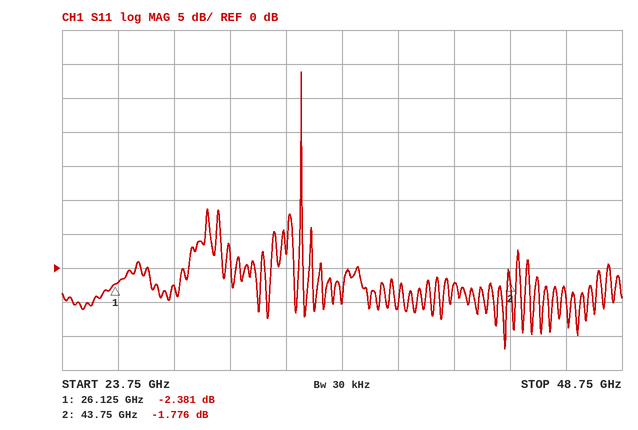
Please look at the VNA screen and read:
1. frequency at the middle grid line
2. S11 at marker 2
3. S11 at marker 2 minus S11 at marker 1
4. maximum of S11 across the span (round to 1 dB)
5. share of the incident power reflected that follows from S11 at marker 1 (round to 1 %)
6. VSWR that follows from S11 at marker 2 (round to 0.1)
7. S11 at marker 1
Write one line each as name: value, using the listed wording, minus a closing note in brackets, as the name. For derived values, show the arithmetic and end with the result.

frequency at the middle grid line: 36.25 GHz
S11 at marker 2: -1.776 dB
S11 at marker 2 minus S11 at marker 1: -1.776 − (-2.381) = 0.605 dB
maximum of S11 across the span: 29 dB
share of the incident power reflected that follows from S11 at marker 1: 10^(-2.381/10) ≈ 58 %
VSWR that follows from S11 at marker 2: (1 + 0.8151)/(1 − 0.8151) ≈ 9.8
S11 at marker 1: -2.381 dB
